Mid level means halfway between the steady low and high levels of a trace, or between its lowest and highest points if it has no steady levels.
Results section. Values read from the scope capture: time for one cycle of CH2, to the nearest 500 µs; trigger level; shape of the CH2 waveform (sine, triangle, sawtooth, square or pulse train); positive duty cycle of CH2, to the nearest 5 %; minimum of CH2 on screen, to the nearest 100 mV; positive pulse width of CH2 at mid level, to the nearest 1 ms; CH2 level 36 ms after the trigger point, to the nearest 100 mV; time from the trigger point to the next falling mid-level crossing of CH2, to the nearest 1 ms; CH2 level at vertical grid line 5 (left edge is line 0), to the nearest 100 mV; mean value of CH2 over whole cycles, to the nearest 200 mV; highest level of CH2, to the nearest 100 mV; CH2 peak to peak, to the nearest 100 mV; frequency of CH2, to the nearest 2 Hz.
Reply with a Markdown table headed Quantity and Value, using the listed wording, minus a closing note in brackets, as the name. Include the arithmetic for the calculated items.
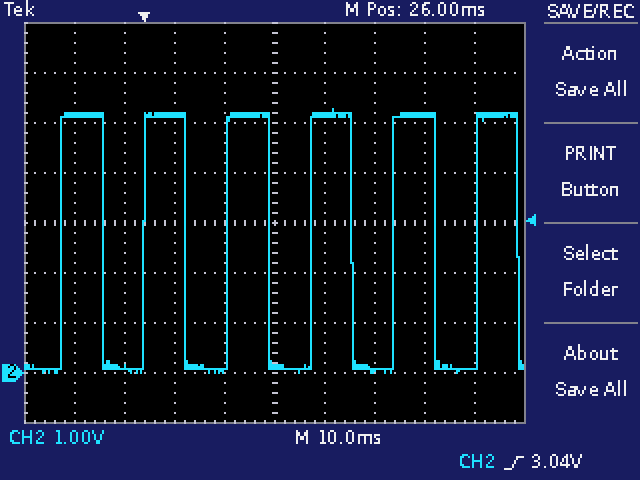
| Quantity | Value |
|---|---|
| time for one cycle of CH2, to the nearest 500 µs | 16.5 ms |
| trigger level | 3.04 V |
| shape of the CH2 waveform | square |
| positive duty cycle of CH2, to the nearest 5 % | 8 ms / 16.5 ms ≈ 48.5 %, so 50 % to the nearest 5 % |
| minimum of CH2 on screen, to the nearest 100 mV | 0.0 V |
| positive pulse width of CH2 at mid level, to the nearest 1 ms | 8 ms |
| CH2 level 36 ms after the trigger point, to the nearest 100 mV | 5.2 V |
| time from the trigger point to the next falling mid-level crossing of CH2, to the nearest 1 ms | 8 ms |
| CH2 level at vertical grid line 5 (left edge is line 0), to the nearest 100 mV | 200 mV |
| mean value of CH2 over whole cycles, to the nearest 200 mV | 0.0 V + 0.5 × (5.3 V − (0.0 V)) ≈ 2.6 V |
| highest level of CH2, to the nearest 100 mV | 5.3 V |
| CH2 peak to peak, to the nearest 100 mV | 5.3 V − (0.0 V) = 5.3 V |
| frequency of CH2, to the nearest 2 Hz | 1 / 16.5 ms ≈ 60.6 Hz, so 60 Hz to the nearest 2 Hz |
